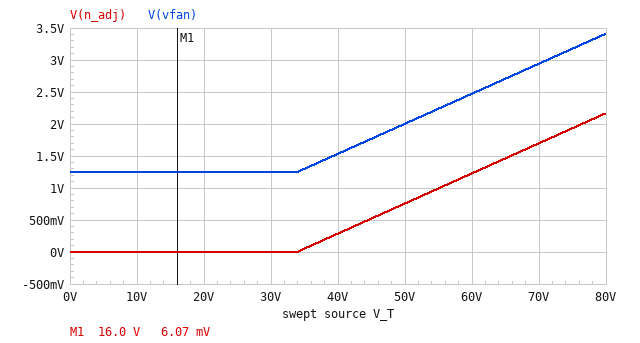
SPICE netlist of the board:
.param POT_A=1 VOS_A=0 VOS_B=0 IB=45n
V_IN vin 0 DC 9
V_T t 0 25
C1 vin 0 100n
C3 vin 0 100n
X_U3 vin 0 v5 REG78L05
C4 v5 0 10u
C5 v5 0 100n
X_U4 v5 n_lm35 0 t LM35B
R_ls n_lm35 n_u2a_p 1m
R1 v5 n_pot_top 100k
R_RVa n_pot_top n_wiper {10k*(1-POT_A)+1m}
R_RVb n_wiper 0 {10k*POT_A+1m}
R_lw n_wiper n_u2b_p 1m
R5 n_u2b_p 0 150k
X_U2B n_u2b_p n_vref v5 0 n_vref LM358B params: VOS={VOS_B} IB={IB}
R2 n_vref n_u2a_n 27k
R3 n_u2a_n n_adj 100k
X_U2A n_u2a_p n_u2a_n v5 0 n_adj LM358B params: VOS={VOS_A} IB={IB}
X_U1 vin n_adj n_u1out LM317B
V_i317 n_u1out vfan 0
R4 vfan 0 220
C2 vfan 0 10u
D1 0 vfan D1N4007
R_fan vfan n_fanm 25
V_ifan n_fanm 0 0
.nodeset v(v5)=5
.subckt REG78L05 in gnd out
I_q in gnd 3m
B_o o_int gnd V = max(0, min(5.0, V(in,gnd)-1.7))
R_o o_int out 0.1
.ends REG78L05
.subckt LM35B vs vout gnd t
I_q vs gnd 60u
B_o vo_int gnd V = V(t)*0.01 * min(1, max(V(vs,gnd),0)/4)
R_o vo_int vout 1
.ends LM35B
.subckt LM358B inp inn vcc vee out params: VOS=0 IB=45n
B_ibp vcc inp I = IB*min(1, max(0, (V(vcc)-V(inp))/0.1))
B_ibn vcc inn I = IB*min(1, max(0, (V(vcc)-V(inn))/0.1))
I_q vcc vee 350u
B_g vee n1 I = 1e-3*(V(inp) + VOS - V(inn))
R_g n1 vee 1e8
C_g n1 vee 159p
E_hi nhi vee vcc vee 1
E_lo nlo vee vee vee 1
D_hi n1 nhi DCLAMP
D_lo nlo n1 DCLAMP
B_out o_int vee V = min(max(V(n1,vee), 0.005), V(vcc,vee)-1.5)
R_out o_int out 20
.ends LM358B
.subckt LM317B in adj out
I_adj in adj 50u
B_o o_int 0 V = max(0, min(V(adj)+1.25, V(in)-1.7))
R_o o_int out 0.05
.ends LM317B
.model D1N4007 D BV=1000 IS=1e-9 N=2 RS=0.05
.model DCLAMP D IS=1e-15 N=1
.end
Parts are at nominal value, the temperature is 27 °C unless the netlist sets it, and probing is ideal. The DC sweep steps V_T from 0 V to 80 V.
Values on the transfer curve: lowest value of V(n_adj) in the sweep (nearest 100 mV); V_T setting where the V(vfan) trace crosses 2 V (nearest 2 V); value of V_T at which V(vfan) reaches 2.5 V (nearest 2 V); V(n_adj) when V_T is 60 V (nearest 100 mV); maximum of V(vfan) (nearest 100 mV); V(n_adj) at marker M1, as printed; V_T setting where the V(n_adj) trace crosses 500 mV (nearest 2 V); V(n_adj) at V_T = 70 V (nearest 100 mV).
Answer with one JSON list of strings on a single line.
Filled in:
["0 V", "50 V", "60 V", "1.2 V", "3.4 V", "6.07 mV", "44 V", "1.7 V"]
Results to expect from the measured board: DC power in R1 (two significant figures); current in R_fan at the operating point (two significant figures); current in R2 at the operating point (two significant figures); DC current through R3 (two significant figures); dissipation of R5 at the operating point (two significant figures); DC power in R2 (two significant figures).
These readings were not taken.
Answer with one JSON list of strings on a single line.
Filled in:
["210 µW", "50 mA", "3.3 µA", "3.3 µA", "1.2 µW", "290 nW"]
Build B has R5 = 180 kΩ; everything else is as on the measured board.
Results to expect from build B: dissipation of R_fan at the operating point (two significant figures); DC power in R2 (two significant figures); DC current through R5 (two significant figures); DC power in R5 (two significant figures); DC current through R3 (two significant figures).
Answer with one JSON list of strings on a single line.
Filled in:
["63 mW", "300 nW", "2.4 µA", "1.0 µW", "3.4 µA"]
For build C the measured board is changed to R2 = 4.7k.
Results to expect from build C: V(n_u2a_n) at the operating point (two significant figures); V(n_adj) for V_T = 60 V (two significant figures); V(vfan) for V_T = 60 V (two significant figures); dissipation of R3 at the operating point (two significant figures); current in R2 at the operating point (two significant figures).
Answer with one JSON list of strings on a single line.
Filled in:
["410 mV", "3.5 V", "4.7 V", "1.6 µW", "4.0 µA"]
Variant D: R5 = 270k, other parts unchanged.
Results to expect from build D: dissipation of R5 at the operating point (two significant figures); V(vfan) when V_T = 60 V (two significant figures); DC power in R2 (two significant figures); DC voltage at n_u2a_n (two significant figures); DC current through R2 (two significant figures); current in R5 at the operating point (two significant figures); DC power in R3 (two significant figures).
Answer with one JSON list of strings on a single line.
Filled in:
["720 nW", "2.4 V", "310 nW", "350 mV", "3.4 µA", "1.6 µA", "1.2 µW"]
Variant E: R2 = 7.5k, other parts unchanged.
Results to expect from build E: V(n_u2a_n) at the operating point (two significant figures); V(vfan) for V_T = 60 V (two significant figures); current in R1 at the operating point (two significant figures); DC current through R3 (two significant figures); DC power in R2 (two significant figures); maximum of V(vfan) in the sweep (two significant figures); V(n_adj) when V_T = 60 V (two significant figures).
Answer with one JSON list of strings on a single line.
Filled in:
["400 mV", "4.1 V", "46 µA", "3.9 µA", "110 nW", "4.7 V", "2.9 V"]
